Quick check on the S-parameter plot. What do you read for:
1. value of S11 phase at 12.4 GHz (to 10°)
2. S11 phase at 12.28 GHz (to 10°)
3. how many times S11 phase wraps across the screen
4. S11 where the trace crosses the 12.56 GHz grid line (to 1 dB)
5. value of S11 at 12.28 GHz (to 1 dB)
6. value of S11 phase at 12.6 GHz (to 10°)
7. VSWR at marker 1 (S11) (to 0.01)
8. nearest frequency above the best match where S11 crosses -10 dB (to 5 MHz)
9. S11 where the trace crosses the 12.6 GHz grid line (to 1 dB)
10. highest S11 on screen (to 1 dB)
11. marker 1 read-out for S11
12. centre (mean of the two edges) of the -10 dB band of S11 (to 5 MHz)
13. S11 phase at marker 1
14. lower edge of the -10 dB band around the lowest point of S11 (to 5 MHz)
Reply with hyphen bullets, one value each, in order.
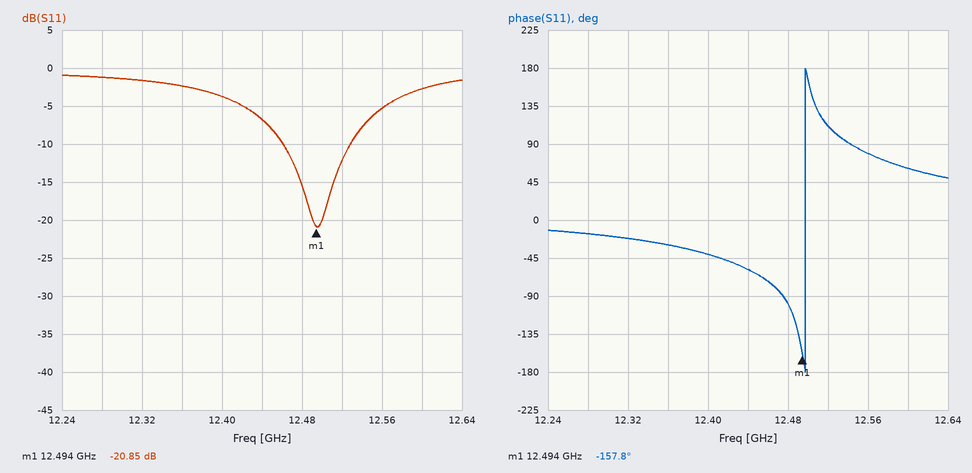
- -40°
- -20°
- 1
- -5 dB
- -1 dB
- 60°
- 1.20
- 12.530 GHz
- -3 dB
- -1 dB
- -20.85 dB
- 12.495 GHz
- -157.8°
- 12.460 GHz
